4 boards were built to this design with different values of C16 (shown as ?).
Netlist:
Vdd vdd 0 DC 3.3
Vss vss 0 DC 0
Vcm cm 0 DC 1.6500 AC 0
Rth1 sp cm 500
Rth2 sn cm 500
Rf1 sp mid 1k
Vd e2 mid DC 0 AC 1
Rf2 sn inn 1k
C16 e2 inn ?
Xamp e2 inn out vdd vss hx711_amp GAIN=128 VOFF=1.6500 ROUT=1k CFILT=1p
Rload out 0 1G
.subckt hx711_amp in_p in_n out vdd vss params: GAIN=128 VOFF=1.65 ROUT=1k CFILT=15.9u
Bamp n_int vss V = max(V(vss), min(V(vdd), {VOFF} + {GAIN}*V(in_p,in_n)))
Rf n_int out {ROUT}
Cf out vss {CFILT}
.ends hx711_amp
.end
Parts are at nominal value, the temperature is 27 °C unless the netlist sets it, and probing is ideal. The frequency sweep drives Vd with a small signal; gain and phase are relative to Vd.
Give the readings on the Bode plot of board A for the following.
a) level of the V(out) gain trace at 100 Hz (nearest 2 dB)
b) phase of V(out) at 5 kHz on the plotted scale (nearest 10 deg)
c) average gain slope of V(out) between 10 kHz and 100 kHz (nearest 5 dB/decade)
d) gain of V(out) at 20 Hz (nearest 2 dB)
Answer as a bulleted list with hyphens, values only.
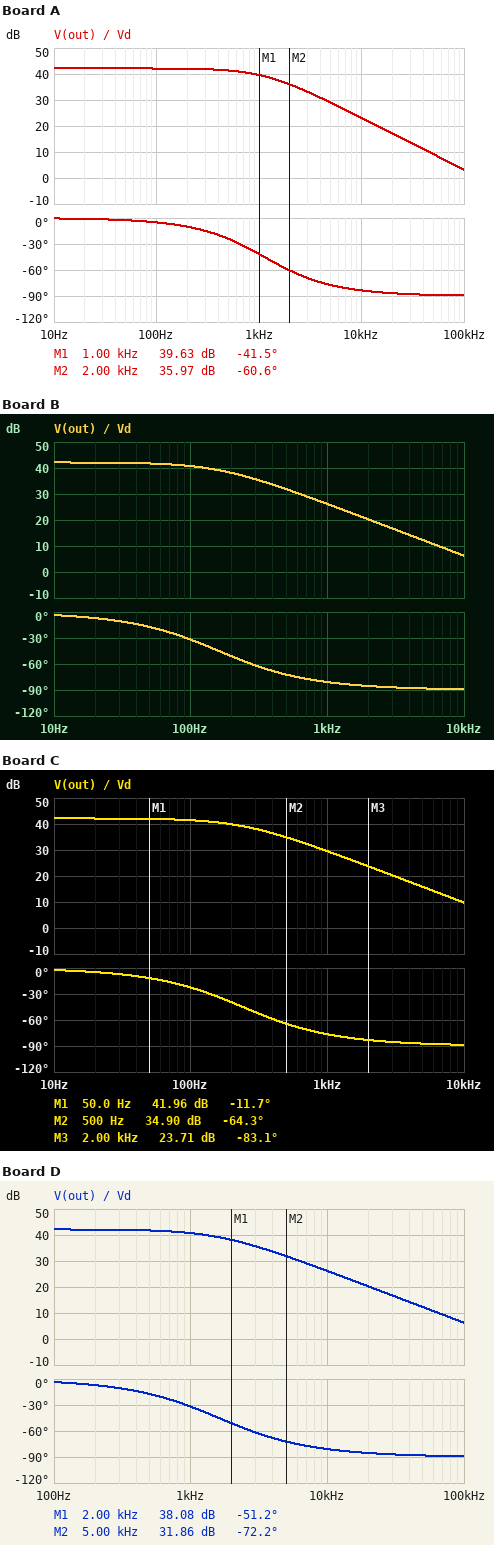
- 42 dB
- -80 deg
- -20 dB/decade
- 42 dB
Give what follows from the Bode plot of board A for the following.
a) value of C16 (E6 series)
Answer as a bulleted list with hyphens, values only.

- 47 nF
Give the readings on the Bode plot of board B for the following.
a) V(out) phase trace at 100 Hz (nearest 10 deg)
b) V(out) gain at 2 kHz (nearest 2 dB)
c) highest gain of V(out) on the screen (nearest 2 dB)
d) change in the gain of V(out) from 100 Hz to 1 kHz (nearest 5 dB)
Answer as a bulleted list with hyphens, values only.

- -30 deg
- 20 dB
- 42 dB
- -15 dB
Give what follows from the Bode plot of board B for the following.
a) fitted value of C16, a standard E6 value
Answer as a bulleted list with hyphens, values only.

- 330 nF
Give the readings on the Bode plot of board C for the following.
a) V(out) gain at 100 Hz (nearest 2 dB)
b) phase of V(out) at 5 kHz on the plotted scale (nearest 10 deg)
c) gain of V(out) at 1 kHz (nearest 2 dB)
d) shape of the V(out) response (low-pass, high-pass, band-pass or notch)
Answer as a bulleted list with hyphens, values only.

- 42 dB
- -90 deg
- 30 dB
- low-pass
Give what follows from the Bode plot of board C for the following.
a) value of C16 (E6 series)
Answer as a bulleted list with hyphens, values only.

- 220 nF
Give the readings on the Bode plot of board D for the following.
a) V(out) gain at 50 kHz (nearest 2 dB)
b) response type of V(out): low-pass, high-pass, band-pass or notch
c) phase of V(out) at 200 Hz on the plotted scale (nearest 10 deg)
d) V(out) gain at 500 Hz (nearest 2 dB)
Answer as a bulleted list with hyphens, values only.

- 12 dB
- low-pass
- -10 deg
- 42 dB
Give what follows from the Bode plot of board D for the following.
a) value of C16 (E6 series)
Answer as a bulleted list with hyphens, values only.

- 33 nF
